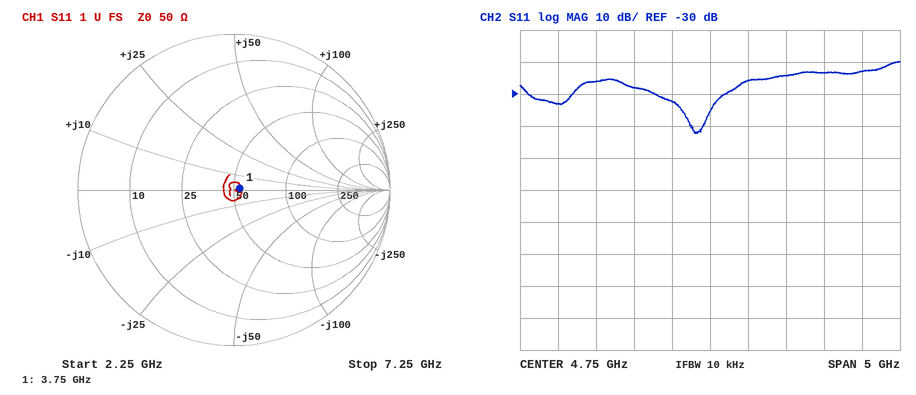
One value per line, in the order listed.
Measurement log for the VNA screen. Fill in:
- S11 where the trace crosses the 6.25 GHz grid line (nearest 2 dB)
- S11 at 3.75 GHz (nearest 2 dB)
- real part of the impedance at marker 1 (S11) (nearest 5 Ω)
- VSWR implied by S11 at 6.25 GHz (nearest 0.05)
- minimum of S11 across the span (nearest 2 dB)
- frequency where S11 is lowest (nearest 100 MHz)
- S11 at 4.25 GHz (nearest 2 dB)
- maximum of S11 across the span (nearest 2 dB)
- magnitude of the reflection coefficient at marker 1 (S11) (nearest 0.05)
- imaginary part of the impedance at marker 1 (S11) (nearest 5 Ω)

-24 dB
-28 dB
55 Ω
1.15
-42 dB
4.6 GHz
-32 dB
-20 dB
0.05
0 Ω
